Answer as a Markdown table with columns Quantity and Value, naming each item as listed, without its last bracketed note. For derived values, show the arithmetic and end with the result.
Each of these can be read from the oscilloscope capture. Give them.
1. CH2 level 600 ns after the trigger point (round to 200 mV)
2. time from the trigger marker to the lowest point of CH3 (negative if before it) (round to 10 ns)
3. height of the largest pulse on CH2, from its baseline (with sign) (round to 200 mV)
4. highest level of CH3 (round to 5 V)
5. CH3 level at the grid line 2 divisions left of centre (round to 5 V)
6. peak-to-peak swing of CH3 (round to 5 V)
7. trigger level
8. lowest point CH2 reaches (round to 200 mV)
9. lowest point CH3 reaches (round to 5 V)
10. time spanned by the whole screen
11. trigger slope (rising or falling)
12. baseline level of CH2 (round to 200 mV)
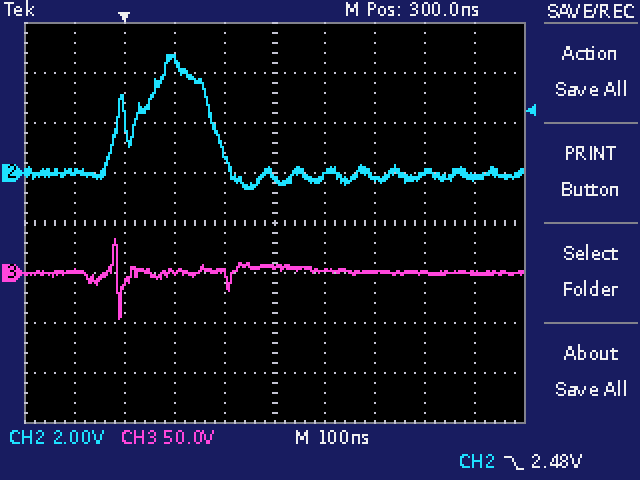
| Quantity | Value |
|---|---|
| CH2 level 600 ns after the trigger point | 0.0 V |
| time from the trigger marker to the lowest point of CH3 (negative if before it) | -10 ns |
| height of the largest pulse on CH2, from its baseline (with sign) | +4.8 V |
| highest level of CH3 | 35 V |
| CH3 level at the grid line 2 divisions left of centre | 0 V |
| peak-to-peak swing of CH3 | 35 V − (-45 V) = 80 V |
| trigger level | 2.48 V |
| lowest point CH2 reaches | -600 mV |
| lowest point CH3 reaches | -45 V |
| time spanned by the whole screen | 1 µs |
| trigger slope | falling |
| baseline level of CH2 | 0.0 V |
